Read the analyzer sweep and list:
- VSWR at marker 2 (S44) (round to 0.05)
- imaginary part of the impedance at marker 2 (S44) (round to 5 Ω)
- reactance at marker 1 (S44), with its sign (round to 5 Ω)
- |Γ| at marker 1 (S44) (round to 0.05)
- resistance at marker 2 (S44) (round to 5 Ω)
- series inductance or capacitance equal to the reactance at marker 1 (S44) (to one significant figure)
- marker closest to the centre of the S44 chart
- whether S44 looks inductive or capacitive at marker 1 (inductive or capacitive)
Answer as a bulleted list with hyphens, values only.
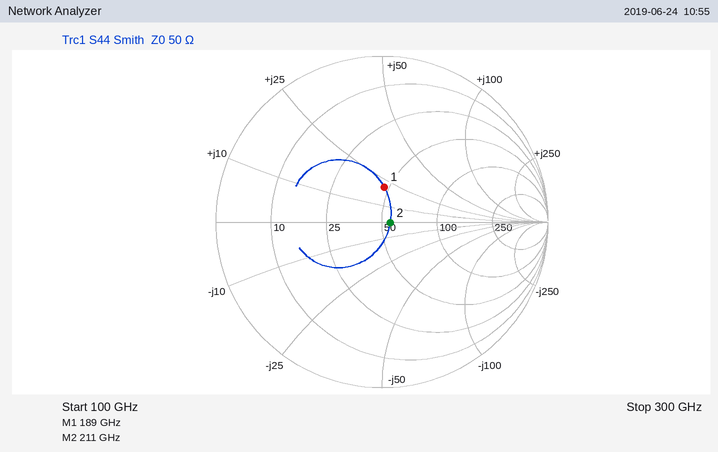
- 1.10
- 0 Ω
- +20 Ω
- 0.20
- 55 Ω
- 20 pH
- marker 2
- inductive
